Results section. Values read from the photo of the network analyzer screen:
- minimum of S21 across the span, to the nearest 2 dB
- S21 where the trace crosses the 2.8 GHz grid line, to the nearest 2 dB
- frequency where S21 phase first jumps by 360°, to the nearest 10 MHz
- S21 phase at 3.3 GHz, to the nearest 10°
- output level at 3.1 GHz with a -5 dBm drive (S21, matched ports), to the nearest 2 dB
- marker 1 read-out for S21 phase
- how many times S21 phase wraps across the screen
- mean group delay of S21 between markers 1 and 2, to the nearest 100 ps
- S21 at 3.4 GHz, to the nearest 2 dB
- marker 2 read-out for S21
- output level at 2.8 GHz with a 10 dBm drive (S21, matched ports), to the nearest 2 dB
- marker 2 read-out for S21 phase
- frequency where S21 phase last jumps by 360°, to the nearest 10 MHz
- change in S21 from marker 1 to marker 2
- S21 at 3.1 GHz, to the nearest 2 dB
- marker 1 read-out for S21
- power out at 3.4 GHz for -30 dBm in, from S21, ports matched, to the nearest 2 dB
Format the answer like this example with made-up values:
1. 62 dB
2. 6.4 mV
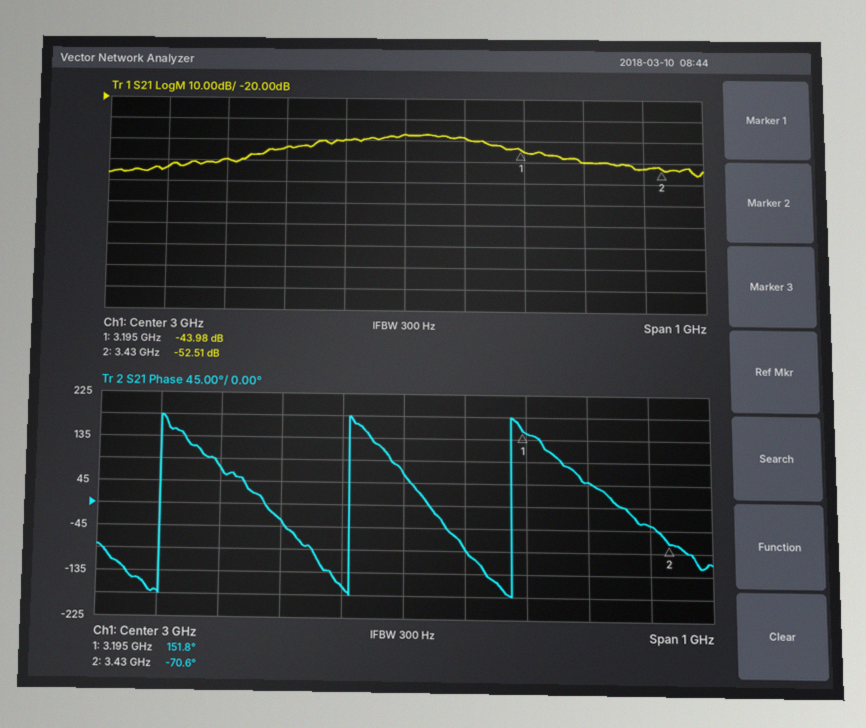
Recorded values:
1. -56 dB
2. -44 dB
3. 2.60 GHz
4. 50°
5. -44 dBm
6. 151.8°
7. 3
8. 2.6 ns
9. -52 dB
10. -52.51 dB
11. -34 dBm
12. -70.6°
13. 3.18 GHz
14. -8.53 dB
15. -38 dB
16. -43.98 dB
17. -82 dBm
